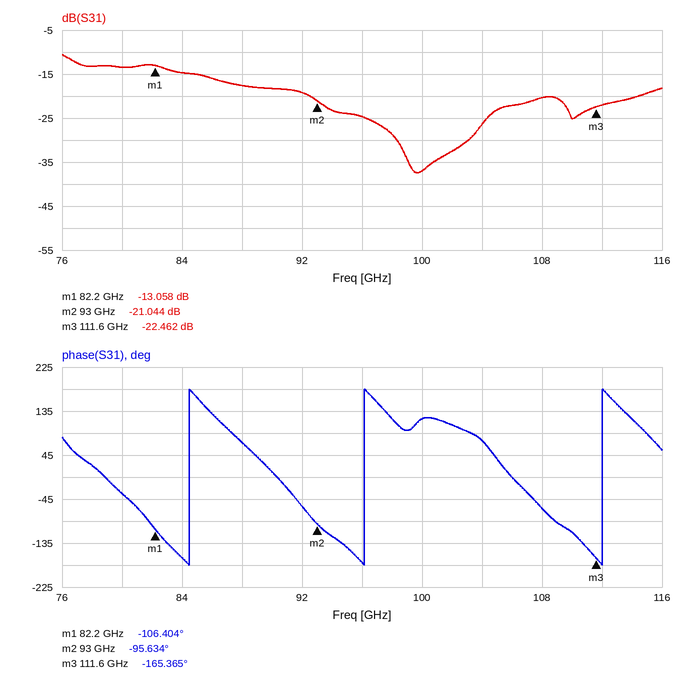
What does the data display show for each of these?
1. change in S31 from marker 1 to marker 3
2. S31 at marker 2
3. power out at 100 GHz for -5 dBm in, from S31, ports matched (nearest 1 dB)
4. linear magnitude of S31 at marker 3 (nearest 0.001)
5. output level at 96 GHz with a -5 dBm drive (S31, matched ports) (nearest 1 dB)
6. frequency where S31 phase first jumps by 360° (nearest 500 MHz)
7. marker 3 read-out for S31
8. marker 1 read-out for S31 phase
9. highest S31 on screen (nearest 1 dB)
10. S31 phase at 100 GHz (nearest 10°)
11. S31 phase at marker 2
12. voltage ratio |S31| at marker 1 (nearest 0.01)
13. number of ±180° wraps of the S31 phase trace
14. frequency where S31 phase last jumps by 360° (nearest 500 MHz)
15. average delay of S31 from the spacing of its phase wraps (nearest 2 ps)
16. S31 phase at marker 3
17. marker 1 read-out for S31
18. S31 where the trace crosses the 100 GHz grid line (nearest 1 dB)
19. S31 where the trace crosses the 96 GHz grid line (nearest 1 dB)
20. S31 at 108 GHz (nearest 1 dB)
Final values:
-9.404 dB
-21.044 dB
-42 dBm
0.075
-30 dBm
84.5 GHz
-22.462 dB
-106.404°
-11 dB
120°
-95.634°
0.22
3
112.0 GHz
72 ps
-165.365°
-13.058 dB
-37 dB
-25 dB
-20 dB
